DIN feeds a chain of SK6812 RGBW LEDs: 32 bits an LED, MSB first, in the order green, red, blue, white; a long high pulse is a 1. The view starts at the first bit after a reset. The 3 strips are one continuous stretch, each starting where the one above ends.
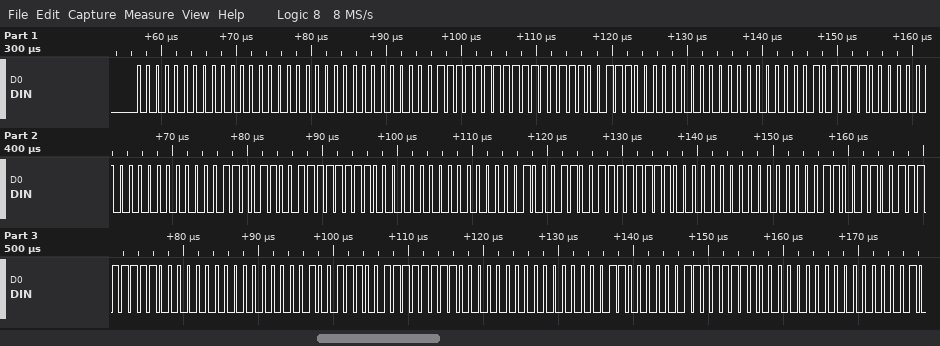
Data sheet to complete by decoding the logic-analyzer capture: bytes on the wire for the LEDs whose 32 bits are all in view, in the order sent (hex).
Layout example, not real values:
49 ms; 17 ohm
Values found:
00 00 00 00 FF FF 38 00 00 BC 00 00 EC FF 00 00 8C FF 00 00 CC FF 00 00 9C FF 00 00 C0 FF 00 00
